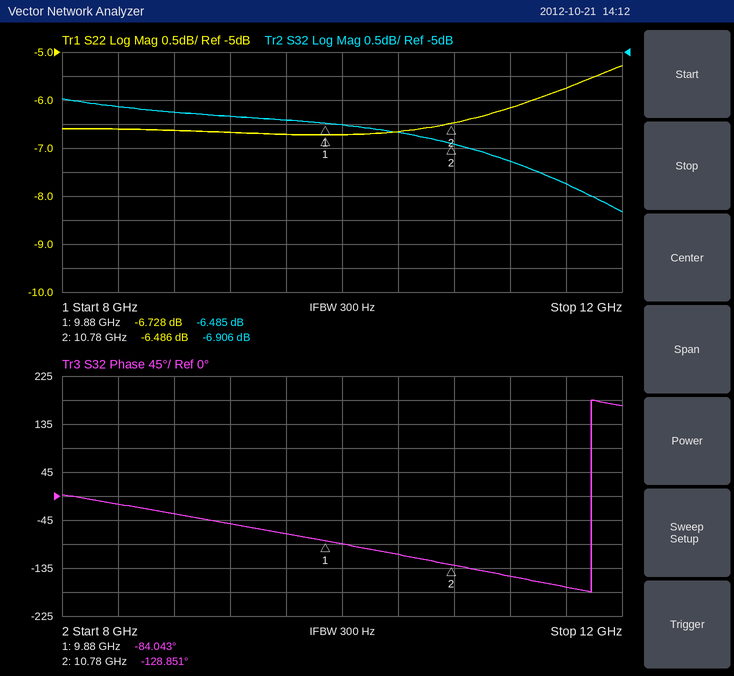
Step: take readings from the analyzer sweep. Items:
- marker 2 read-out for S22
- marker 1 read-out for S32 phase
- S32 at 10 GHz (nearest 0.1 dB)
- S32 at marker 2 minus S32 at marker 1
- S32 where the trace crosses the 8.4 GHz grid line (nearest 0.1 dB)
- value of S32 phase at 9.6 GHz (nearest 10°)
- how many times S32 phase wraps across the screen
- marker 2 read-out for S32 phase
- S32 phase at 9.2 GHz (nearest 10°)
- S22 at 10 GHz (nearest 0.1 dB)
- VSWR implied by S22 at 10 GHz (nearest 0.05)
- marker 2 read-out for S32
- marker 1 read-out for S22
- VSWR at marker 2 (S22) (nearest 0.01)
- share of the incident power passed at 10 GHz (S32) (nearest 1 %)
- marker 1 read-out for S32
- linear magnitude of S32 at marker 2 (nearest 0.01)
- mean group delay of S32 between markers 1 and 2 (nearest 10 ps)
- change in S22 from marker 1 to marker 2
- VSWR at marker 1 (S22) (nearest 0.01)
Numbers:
-6.486 dB
-84.043°
-6.5 dB
-0.421 dB
-6.1 dB
-70°
1
-128.851°
-50°
-6.7 dB
2.70
-6.906 dB
-6.728 dB
2.80
22 %
-6.485 dB
0.45
140 ps
0.242 dB
2.71
